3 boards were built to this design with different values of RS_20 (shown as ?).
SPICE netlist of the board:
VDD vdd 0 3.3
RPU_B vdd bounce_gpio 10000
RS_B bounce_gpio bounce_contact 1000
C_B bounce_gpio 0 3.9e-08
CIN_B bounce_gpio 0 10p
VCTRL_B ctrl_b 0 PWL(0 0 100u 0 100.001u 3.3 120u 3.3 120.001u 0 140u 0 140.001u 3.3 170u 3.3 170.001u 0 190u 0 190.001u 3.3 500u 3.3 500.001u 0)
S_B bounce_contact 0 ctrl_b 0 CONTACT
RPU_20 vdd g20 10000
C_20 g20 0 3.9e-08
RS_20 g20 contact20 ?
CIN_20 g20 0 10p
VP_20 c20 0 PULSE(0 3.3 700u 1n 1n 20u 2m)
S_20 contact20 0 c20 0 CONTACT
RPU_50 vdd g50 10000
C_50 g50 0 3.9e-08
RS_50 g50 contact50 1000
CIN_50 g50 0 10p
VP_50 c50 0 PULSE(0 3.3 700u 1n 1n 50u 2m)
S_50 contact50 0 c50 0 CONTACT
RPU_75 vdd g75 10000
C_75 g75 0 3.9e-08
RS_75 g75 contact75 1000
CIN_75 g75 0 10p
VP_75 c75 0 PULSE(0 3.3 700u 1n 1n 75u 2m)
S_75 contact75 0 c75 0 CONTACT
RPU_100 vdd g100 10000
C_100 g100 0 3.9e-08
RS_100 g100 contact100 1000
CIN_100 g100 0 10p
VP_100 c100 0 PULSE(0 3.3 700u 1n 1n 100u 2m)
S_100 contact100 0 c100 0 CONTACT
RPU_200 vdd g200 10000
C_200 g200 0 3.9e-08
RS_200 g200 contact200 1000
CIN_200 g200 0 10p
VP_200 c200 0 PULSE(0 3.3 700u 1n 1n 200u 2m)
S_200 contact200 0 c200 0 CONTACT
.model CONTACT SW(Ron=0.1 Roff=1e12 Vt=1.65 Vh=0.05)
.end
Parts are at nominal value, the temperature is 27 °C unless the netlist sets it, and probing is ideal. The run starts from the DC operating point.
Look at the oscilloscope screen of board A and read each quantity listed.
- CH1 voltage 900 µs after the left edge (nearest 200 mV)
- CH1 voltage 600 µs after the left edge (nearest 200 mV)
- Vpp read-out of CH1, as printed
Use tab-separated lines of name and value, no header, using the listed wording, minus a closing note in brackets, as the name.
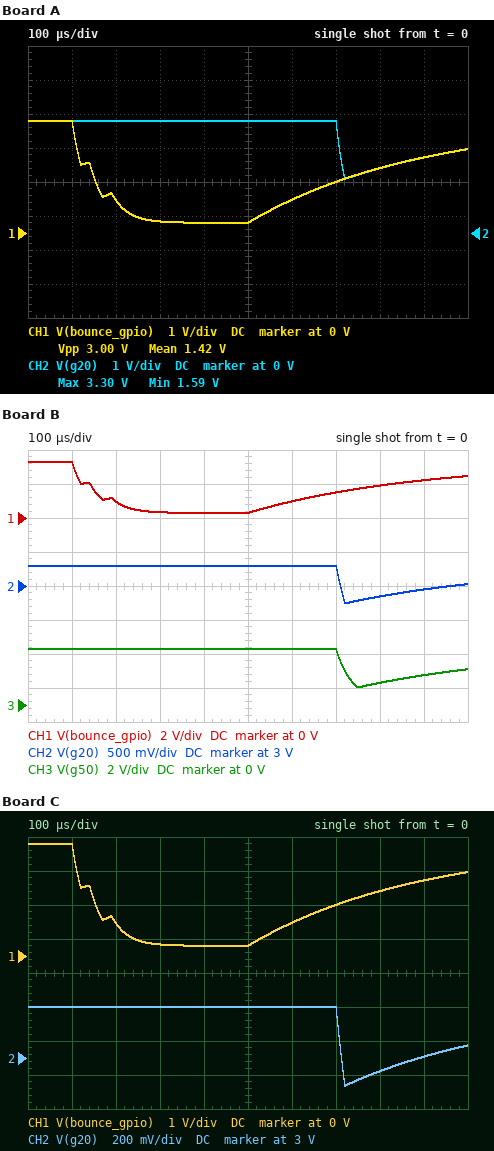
CH1 voltage 900 µs after the left edge	2.2 V
CH1 voltage 600 µs after the left edge	1.0 V
Vpp read-out of CH1, as printed	3.00 V
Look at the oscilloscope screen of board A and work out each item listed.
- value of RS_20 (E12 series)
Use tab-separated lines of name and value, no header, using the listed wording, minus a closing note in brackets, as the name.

value of RS_20	680 Ω
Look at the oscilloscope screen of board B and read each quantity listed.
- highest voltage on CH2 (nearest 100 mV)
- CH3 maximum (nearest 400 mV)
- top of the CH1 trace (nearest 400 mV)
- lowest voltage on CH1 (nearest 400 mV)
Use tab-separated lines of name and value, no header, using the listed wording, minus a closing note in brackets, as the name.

highest voltage on CH2	3.3 V
CH3 maximum	3.2 V
top of the CH1 trace	3.2 V
lowest voltage on CH1	400 mV
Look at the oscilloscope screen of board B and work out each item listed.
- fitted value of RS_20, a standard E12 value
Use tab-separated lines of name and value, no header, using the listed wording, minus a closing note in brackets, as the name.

fitted value of RS_20, a standard E12 value	2.7 kΩ
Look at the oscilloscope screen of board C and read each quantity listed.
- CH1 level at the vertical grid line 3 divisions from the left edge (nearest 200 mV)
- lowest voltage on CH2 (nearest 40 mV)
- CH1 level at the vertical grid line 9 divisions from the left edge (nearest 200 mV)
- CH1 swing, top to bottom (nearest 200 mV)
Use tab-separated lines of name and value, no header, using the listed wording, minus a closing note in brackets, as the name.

CH1 level at the vertical grid line 3 divisions from the left edge	400 mV
lowest voltage on CH2	2.84 V
CH1 level at the vertical grid line 9 divisions from the left edge	2.2 V
CH1 swing, top to bottom	3.0 V
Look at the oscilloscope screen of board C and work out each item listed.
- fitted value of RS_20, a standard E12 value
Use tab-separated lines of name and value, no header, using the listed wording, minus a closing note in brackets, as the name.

fitted value of RS_20, a standard E12 value	3.3 kΩ
